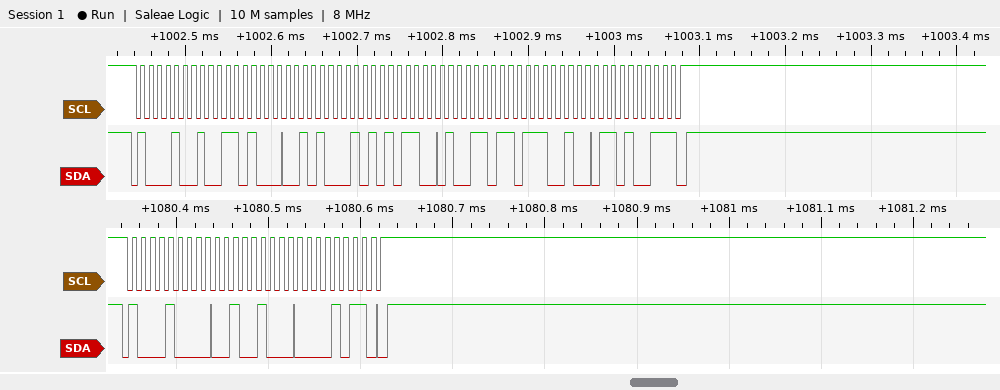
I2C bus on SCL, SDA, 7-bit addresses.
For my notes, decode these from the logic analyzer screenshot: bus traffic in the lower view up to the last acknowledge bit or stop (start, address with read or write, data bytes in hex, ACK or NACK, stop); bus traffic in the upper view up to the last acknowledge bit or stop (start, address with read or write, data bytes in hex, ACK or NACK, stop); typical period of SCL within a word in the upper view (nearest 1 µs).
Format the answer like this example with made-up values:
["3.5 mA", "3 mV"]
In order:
["start, address 44 write ACK, 24 ACK, 0B ACK, stop", "start, address 44 read ACK, 68 ACK, 51 ACK, AC ACK, 9B ACK, E4 ACK, D3 NACK, stop", "10 µs"]
